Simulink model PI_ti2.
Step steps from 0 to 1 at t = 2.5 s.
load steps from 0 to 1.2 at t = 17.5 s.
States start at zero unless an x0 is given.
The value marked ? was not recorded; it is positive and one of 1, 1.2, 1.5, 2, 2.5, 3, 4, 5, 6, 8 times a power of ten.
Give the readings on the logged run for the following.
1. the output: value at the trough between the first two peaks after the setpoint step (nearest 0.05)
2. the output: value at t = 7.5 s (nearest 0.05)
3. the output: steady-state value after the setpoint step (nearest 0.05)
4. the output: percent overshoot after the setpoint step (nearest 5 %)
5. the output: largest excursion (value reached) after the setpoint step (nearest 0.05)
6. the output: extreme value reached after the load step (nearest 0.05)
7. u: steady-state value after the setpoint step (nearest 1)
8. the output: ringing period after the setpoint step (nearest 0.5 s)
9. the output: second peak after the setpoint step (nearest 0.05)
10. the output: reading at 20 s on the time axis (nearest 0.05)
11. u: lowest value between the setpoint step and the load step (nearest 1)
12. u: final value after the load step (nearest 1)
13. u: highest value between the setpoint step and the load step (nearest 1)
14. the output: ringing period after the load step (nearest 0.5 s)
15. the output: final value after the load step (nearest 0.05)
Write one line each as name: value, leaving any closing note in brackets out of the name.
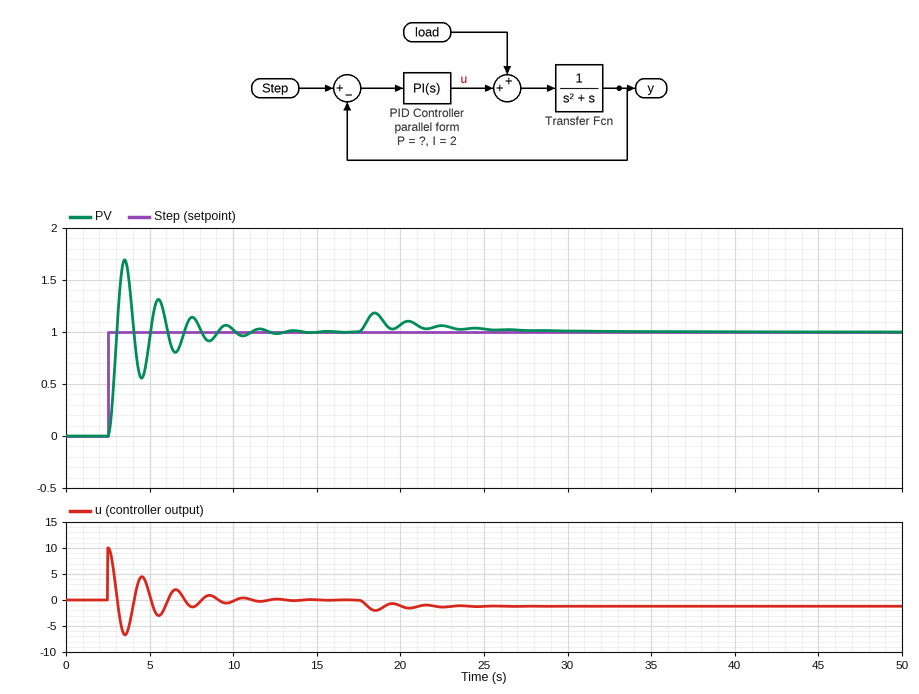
the output: value at the trough between the first two peaks after the setpoint step: 0.55
the output: value at t = 7.5 s: 1.15
the output: steady-state value after the setpoint step: 1.00
the output: percent overshoot after the setpoint step: 70 %
the output: largest excursion (value reached) after the setpoint step: 1.70
the output: extreme value reached after the load step: 1.20
u: steady-state value after the setpoint step: 0
the output: ringing period after the setpoint step: 2.0 s
the output: second peak after the setpoint step: 1.30
the output: reading at 20 s on the time axis: 1.05
u: lowest value between the setpoint step and the load step: -7
u: final value after the load step: -1
u: highest value between the setpoint step and the load step: 10
the output: ringing period after the load step: 2.0 s
the output: final value after the load step: 1.00
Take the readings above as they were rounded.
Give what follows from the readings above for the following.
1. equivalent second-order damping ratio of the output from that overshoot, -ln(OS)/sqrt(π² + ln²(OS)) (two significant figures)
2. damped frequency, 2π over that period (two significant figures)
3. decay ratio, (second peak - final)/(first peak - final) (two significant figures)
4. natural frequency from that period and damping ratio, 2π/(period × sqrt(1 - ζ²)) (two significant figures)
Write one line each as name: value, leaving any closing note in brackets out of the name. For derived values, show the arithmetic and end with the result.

equivalent second-order damping ratio of the output from that overshoot, -ln(OS)/sqrt(π² + ln²(OS)): ln(0.7) = -0.357; 0.357 / sqrt(9.870 + 0.127) = 0.11
damped frequency, 2π over that period: 2π / 2 = 3.1 rad/s
decay ratio, (second peak - final)/(first peak - final): (1.3 - 1) / (1.7 - 1) = 0.43
natural frequency from that period and damping ratio, 2π/(period × sqrt(1 - ζ²)): 2π / (2 × sqrt(1 - 0.11²)) = 3.2 rad/s
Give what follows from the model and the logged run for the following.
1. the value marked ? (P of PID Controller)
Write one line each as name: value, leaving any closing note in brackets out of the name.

the value marked ?: 10
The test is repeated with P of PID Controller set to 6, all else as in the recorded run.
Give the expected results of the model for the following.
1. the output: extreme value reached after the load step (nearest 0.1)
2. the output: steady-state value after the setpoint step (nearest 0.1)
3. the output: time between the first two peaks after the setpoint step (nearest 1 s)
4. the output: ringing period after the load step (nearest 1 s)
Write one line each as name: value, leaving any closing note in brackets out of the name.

the output: extreme value reached after the load step: 1.3
the output: steady-state value after the setpoint step: 1.0
the output: time between the first two peaks after the setpoint step: 3 s
the output: ringing period after the load step: 3 s
